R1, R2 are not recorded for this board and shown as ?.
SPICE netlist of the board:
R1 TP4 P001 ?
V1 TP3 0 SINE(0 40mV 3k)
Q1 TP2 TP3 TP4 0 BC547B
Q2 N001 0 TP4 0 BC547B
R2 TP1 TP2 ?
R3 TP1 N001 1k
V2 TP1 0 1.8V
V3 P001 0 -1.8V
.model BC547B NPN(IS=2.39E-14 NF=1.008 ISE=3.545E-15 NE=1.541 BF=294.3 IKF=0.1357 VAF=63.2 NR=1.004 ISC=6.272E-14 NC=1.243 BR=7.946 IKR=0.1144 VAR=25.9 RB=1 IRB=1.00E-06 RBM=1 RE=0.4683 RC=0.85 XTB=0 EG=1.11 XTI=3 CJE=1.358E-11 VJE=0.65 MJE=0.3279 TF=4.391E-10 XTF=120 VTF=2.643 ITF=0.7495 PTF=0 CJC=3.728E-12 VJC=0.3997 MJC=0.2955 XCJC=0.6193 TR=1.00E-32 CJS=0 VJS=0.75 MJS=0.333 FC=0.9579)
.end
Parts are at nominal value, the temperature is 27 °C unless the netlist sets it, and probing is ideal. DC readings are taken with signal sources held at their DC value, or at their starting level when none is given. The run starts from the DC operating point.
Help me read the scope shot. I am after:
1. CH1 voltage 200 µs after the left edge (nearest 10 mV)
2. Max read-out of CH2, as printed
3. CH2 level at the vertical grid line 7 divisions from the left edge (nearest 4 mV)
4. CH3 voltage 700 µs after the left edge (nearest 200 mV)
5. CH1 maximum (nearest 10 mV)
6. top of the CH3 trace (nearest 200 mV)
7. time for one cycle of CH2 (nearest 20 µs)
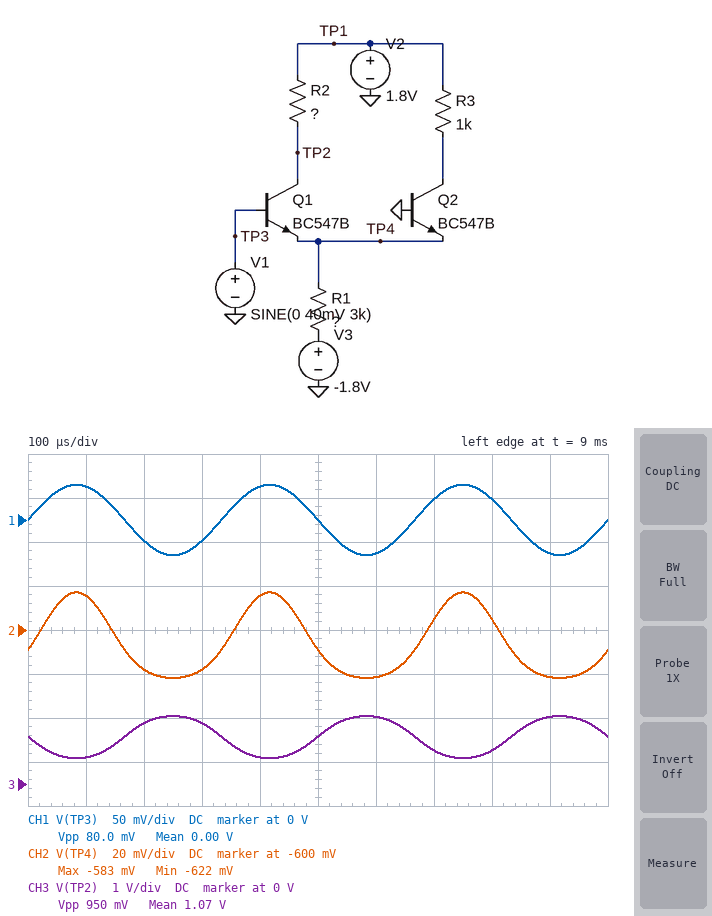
-20 mV
-583 mV
-596 mV
800 mV
40 mV
1.6 V
340 µs
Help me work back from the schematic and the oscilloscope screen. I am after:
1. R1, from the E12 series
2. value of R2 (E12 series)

1.8 kΩ
2.2 kΩ
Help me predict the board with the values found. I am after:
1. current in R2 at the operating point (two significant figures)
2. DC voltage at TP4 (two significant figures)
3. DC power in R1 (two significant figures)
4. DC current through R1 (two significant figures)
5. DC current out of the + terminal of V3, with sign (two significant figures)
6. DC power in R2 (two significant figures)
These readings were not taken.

330 µA
-610 mV
790 µW
660 µA
-660 µA
240 µW
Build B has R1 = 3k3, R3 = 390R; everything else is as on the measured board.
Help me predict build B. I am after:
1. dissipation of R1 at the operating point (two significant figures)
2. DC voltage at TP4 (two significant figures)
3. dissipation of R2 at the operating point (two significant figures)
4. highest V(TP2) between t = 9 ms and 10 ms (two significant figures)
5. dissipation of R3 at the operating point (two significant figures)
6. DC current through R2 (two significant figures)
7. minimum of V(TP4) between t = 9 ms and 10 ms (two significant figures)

440 µW
-590 mV
73 µW
1.7 V
13 µW
180 µA
-610 mV
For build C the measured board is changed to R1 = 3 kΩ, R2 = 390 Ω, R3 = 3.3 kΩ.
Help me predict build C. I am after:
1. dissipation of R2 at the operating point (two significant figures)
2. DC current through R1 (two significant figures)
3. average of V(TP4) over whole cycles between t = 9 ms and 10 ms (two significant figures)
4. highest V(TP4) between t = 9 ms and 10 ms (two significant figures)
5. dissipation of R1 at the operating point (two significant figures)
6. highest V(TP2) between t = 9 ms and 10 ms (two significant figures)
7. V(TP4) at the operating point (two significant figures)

16 µW
400 µA
-590 mV
-570 mV
480 µW
1.8 V
-600 mV
